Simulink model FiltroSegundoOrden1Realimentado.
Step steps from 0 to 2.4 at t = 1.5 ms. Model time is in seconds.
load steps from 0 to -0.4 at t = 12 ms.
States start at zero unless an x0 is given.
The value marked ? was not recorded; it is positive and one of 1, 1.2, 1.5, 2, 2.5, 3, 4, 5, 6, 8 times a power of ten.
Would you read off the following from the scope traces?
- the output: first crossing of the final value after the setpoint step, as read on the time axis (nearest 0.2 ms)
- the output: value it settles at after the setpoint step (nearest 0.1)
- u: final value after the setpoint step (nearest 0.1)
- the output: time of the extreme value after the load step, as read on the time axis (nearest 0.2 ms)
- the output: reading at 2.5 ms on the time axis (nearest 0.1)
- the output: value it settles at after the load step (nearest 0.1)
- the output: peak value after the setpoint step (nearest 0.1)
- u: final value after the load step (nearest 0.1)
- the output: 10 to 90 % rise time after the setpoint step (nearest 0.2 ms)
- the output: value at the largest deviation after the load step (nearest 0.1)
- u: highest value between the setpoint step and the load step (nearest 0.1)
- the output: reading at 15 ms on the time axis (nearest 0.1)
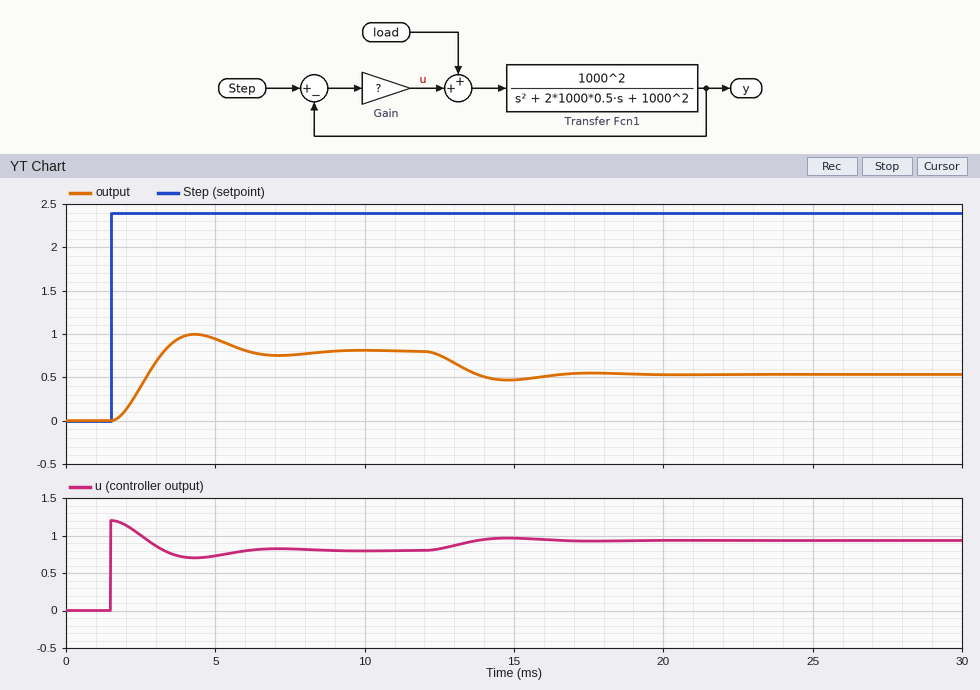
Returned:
3.2 ms
0.8
0.8
14.8 ms
0.4
0.5
1.0
0.9
1.2 ms
0.5
1.2
0.5
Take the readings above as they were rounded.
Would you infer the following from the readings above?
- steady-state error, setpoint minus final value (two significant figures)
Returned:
1.6
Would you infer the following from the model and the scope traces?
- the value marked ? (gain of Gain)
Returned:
0.5
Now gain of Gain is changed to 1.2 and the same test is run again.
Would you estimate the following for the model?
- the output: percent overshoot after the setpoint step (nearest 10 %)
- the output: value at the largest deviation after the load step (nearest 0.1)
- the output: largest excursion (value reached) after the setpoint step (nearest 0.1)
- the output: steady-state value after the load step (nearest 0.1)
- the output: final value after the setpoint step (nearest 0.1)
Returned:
30 %
1.1
1.7
1.1
1.3
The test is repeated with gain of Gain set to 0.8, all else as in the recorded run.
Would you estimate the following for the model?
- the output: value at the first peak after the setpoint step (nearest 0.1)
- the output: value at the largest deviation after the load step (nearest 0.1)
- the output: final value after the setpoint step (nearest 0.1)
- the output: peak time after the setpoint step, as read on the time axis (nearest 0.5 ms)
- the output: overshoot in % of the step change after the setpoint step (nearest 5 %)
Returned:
1.4
0.8
1.1
4.0 ms
30 %
